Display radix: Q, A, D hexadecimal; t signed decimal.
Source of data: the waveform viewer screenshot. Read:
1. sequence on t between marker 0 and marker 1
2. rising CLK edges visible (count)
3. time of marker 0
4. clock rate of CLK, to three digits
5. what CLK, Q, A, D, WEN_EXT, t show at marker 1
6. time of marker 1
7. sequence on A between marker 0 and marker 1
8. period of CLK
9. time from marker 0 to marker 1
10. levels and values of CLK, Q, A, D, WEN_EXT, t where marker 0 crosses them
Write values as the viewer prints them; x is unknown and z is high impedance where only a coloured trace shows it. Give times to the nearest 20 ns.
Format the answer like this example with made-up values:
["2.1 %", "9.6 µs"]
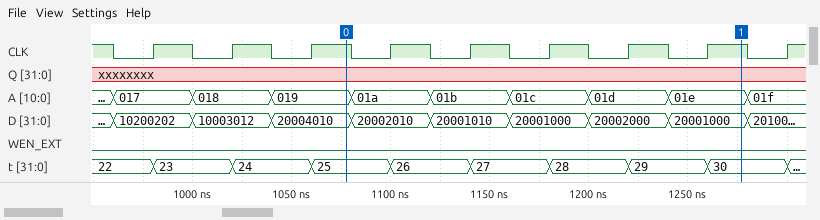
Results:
["25, 26, 27, 28, 29, 30", "9", "1080 ns", "25.0 MHz", "CLK=1, Q=xxxxxxxx, A=01e, D=20001000, WEN_EXT=0, t=30", "1280 ns", "019, 01a, 01b, 01c, 01d, 01e", "40 ns", "200 ns", "CLK=1, Q=xxxxxxxx, A=019, D=20004010, WEN_EXT=0, t=25"]
